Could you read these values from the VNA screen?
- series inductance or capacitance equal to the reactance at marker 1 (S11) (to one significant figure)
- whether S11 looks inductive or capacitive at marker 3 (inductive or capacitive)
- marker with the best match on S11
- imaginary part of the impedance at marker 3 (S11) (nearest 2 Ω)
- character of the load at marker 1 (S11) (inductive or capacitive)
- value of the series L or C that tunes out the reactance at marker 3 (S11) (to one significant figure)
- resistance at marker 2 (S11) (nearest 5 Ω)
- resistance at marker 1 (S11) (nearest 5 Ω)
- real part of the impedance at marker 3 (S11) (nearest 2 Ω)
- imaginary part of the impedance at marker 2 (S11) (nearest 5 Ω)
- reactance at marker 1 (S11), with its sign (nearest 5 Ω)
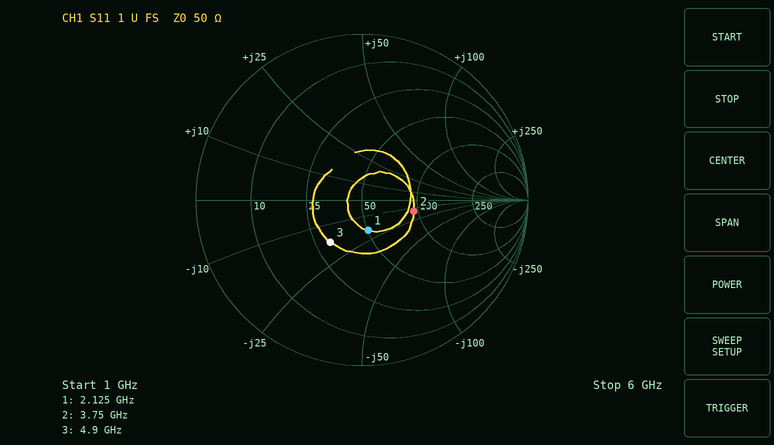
4 pF
capacitive
marker 1
-18 Ω
capacitive
600 pH
95 Ω
50 Ω
30 Ω
-15 Ω
-20 Ω
